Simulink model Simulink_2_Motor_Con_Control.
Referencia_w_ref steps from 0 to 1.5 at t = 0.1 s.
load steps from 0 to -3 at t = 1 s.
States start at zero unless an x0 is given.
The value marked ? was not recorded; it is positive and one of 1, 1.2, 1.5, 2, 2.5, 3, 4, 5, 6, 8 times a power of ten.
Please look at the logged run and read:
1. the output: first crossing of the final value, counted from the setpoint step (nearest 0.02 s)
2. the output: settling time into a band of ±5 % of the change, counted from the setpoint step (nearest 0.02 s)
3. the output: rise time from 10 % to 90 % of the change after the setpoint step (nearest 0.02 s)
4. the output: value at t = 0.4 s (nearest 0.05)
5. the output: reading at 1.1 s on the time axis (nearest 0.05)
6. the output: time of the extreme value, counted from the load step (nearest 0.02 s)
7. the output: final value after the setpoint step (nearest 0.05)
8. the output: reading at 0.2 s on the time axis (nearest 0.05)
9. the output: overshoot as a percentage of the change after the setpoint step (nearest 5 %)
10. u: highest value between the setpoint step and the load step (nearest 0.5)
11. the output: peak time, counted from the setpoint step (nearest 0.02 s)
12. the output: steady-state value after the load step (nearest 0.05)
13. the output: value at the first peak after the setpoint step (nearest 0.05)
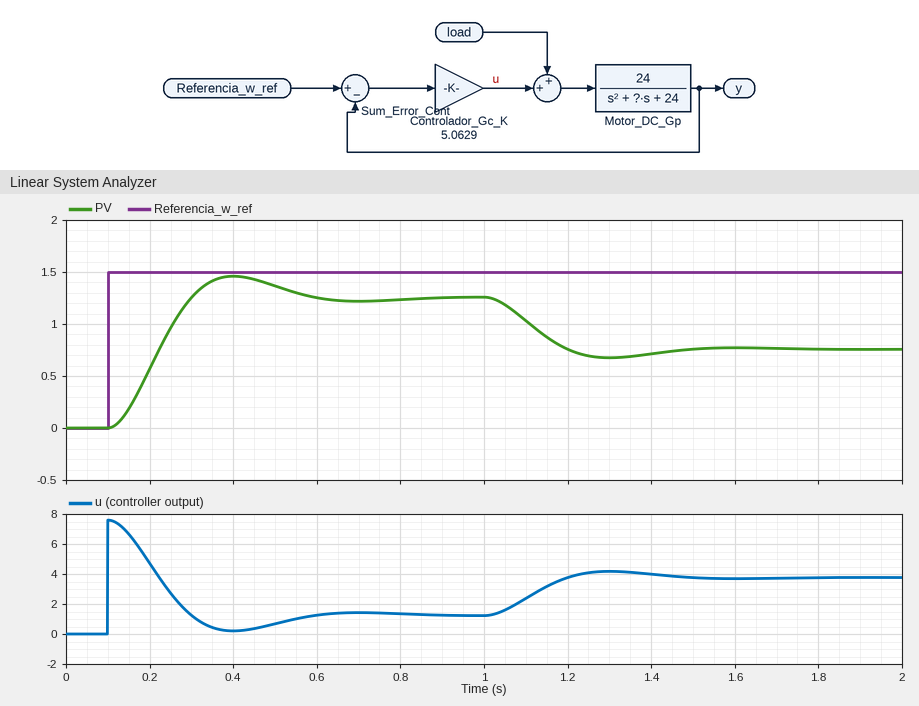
0.20 s
0.44 s
0.14 s
1.45
1.05
0.30 s
1.25
0.55
15 %
7.5
0.30 s
0.75
1.45
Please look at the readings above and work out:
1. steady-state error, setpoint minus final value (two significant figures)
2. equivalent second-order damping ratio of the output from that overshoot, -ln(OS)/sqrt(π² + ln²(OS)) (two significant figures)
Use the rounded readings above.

0.25
0.52
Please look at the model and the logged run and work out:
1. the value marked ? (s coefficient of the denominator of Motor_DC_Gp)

12
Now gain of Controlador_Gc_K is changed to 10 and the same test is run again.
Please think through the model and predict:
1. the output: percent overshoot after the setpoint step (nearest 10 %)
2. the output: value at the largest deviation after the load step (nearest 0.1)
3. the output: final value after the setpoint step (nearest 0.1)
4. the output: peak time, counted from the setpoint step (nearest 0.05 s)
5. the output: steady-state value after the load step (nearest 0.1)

30 %
1.0
1.4
0.20 s
1.1
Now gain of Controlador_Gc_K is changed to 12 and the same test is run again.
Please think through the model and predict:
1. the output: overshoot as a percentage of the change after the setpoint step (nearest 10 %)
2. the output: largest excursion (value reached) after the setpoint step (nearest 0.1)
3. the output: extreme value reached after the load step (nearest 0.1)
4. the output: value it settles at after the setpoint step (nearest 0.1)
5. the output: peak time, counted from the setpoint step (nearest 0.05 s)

30 %
1.8
1.1
1.4
0.20 s
